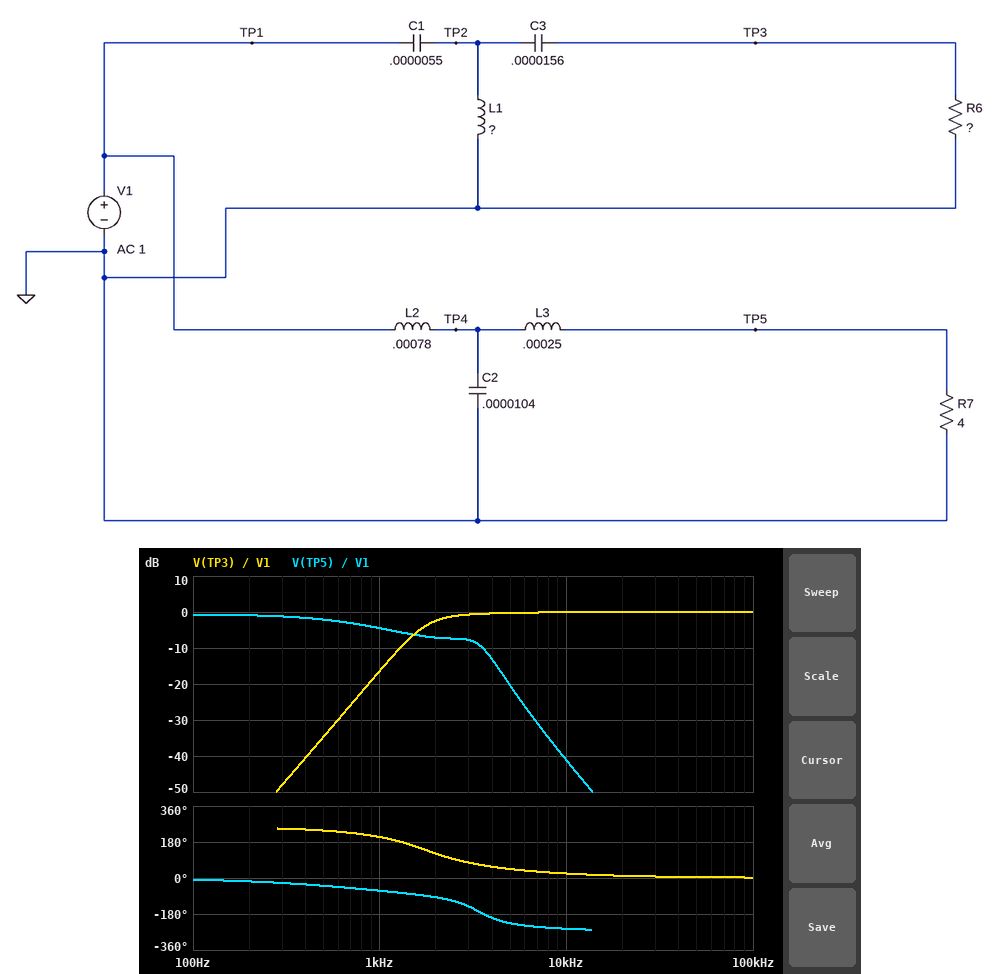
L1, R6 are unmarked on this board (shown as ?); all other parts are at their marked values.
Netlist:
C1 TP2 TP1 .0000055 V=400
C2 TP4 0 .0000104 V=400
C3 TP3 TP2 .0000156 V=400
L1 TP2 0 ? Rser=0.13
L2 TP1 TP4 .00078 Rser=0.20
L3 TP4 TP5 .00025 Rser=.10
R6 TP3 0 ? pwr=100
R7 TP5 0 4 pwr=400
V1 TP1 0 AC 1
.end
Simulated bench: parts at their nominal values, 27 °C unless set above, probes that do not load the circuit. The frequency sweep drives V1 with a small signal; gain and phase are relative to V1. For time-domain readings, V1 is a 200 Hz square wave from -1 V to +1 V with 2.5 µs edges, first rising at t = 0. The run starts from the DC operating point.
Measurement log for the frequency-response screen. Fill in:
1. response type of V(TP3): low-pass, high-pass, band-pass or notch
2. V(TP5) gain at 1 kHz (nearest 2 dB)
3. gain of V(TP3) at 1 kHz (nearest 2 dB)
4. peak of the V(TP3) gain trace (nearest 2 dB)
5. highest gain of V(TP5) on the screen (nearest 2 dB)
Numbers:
high-pass
-4 dB
-16 dB
0 dB
0 dB
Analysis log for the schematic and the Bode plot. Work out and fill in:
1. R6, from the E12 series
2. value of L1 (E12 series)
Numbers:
10 Ω
680 µH
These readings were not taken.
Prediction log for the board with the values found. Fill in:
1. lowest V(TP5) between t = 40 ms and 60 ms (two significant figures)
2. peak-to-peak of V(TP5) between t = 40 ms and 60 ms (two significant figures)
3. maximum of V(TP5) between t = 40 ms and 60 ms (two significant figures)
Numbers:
-930 mV
1.9 V
930 mV
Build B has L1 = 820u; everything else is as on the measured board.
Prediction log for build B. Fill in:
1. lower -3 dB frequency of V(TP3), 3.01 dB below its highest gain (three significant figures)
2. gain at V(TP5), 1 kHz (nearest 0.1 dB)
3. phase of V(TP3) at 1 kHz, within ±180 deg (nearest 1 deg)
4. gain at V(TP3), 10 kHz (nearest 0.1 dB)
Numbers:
1.82 kHz
-4.5 dB
-161 deg
-0.2 dB
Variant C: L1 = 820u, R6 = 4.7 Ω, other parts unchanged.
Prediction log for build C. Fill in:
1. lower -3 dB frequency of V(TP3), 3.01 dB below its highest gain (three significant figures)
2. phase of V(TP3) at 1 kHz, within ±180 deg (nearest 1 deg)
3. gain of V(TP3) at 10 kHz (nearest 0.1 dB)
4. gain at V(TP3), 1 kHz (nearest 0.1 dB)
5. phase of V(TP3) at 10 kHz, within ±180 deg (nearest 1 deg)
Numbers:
7.42 kHz
-143 deg
-1.9 dB
-15.8 dB
41 deg
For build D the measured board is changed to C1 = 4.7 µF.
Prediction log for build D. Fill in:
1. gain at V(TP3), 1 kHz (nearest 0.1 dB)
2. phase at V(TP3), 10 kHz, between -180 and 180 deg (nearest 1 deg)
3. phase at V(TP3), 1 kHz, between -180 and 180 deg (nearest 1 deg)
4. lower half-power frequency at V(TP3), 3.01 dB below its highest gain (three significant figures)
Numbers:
-18.0 dB
25 deg
-154 deg
2.21 kHz
